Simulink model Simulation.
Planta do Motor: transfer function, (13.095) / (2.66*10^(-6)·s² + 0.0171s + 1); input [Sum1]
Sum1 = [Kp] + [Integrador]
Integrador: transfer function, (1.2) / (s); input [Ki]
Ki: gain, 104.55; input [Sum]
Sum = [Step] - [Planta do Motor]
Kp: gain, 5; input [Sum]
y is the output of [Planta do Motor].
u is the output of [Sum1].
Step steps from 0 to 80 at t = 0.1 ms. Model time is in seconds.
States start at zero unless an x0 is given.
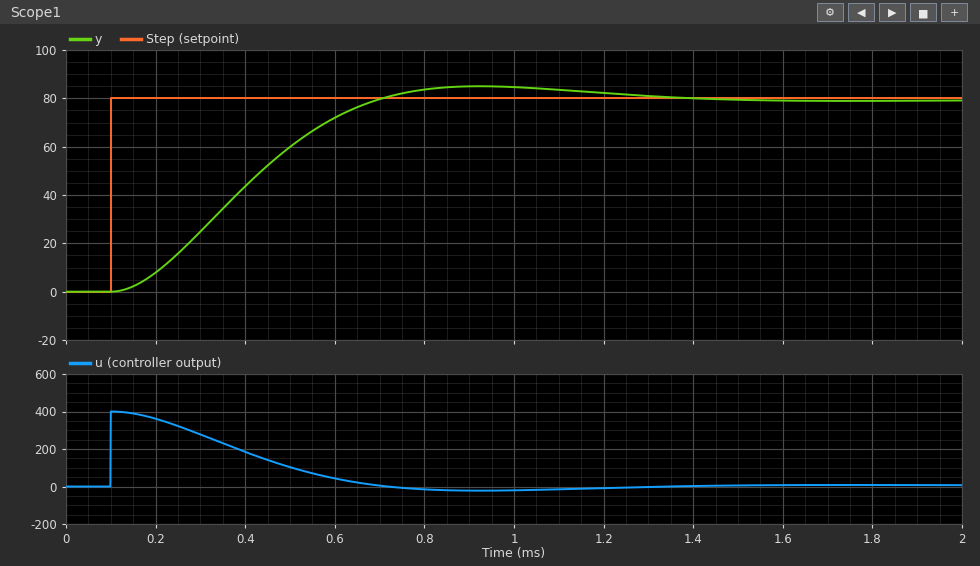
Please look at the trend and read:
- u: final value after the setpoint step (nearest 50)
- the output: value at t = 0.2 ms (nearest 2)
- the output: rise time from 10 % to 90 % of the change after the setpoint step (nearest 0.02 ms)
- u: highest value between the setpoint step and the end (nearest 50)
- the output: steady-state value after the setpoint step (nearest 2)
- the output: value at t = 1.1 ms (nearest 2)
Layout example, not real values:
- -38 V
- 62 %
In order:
- 0
- 8
- 0.40 ms
- 400
- 80
- 84
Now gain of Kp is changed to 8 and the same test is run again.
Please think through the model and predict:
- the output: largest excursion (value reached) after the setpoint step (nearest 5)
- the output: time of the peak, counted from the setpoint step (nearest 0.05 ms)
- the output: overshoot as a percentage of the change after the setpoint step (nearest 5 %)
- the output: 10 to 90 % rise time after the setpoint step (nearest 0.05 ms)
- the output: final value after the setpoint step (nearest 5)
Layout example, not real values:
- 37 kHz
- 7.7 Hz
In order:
- 90
- 0.60 ms
- 15 %
- 0.25 ms
- 80
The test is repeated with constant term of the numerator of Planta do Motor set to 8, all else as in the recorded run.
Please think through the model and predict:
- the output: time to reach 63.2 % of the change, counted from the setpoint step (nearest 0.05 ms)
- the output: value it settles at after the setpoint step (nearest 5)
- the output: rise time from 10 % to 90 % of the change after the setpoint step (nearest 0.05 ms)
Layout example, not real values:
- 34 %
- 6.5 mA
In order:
- 0.50 ms
- 80
- 0.65 ms
